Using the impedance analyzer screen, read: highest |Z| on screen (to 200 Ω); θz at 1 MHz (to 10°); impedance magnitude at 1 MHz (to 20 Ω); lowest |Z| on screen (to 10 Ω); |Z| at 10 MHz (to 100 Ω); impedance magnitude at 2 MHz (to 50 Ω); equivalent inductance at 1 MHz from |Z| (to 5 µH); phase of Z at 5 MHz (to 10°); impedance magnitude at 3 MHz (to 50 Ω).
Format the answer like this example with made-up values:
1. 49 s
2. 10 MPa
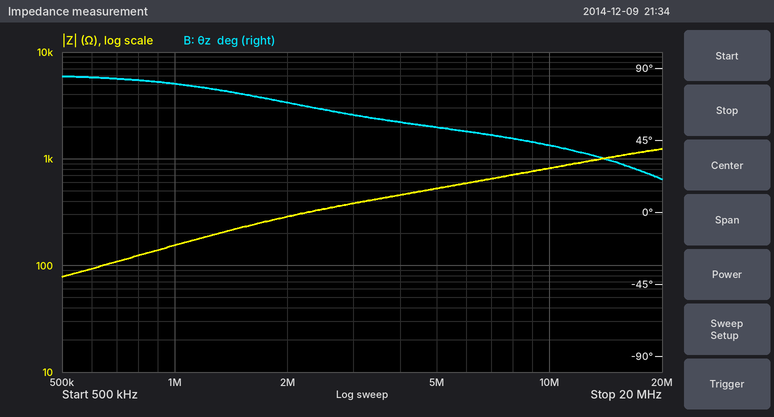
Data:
1. 1.2 kΩ
2. 80°
3. 160 Ω
4. 80 Ω
5. 800 Ω
6. 300 Ω
7. 25 µH
8. 50°
9. 400 Ω
